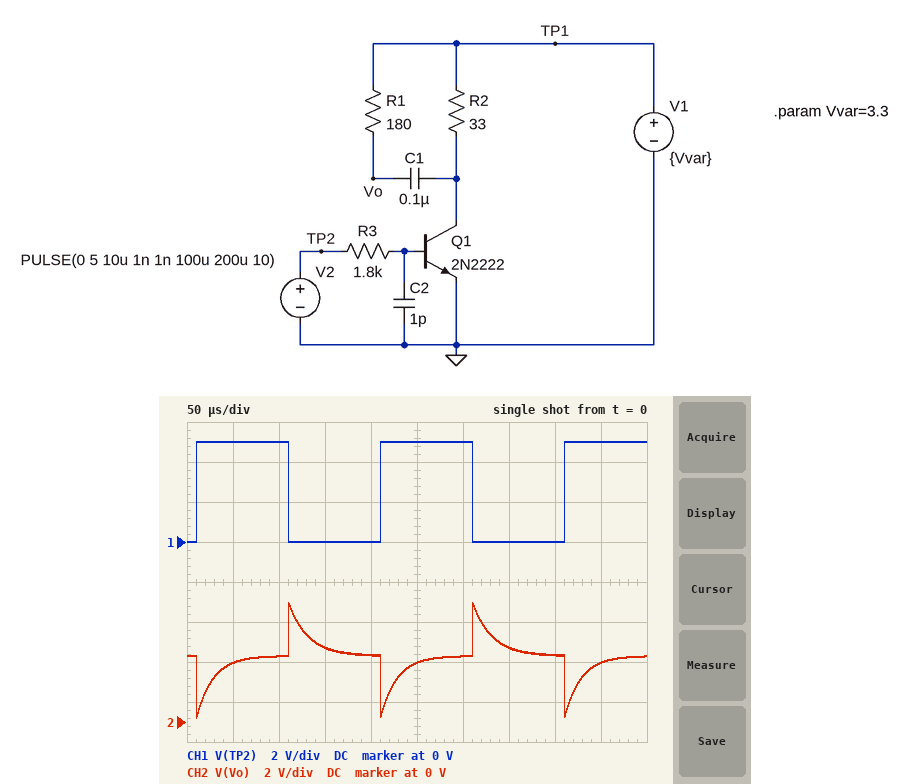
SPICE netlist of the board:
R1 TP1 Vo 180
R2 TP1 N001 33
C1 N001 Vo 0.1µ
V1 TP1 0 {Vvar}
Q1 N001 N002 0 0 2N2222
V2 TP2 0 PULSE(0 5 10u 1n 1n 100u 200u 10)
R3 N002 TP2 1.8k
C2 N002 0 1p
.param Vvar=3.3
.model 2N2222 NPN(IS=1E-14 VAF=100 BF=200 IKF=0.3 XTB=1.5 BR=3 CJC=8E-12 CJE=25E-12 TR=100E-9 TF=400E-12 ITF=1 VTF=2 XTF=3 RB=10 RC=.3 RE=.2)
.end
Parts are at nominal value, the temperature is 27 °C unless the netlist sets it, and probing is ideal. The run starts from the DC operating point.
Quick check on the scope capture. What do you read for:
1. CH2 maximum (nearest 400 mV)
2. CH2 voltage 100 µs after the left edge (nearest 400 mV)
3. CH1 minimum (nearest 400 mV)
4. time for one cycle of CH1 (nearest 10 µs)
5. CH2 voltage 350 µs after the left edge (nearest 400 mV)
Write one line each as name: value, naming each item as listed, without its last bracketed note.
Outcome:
CH2 maximum: 6.0 V
CH2 voltage 100 µs after the left edge: 3.2 V
CH1 minimum: 0 V
time for one cycle of CH1: 200 µs
CH2 voltage 350 µs after the left edge: 3.6 V
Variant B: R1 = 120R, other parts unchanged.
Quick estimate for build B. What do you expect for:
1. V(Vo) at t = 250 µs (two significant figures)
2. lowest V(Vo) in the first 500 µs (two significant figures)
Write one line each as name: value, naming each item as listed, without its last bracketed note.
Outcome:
V(Vo) at t = 250 µs: 3.2 V
lowest V(Vo) in the first 500 µs: 220 mV
